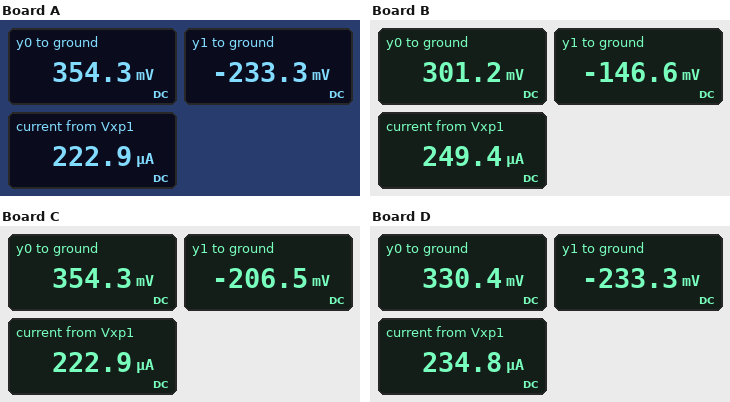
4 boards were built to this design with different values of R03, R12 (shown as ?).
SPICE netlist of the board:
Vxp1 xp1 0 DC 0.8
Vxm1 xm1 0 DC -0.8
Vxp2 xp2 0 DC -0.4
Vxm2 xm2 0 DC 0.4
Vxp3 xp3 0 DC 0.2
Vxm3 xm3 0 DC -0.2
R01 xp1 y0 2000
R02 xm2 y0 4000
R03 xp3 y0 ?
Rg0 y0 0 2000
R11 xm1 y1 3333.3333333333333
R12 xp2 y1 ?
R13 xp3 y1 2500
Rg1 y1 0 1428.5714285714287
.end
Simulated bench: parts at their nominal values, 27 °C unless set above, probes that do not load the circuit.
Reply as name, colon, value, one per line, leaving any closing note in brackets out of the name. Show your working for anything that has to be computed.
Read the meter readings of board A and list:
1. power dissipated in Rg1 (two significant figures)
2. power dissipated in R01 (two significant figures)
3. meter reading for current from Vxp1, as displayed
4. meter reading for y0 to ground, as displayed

power dissipated in Rg1: (0 V - (-233.3 mV))^2 / 1.429 kΩ = 38 µW
power dissipated in R01: (800 mV - 354.3 mV)^2 / 2 kΩ = 99 µW
meter reading for current from Vxp1, as displayed: 222.9 µA
meter reading for y0 to ground, as displayed: 354.3 mV
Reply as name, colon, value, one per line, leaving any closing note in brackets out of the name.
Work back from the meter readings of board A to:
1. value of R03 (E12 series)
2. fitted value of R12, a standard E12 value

value of R03: 2.7 kΩ
fitted value of R12, a standard E12 value: 1 kΩ
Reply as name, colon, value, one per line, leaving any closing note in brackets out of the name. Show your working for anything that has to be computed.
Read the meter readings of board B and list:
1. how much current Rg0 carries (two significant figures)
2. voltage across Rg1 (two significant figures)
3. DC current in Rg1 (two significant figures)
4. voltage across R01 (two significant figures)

how much current Rg0 carries: (301.2 mV) / 2 kΩ = 150 µA
voltage across Rg1: 0 V - (-146.6 mV) = 150 mV
DC current in Rg1: (0 V - (-146.6 mV)) / 1.429 kΩ = 100 µA
voltage across R01: 800 mV - 301.2 mV = 500 mV
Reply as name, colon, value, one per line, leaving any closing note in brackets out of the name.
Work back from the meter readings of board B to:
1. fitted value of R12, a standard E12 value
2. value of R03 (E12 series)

fitted value of R12, a standard E12 value: 5.6 kΩ
value of R03: 820 Ω
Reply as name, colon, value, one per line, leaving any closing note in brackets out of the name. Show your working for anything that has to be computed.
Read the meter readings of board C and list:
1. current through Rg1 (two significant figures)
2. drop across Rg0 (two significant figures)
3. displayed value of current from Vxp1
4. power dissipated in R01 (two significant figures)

current through Rg1: (0 V - (-206.5 mV)) / 1.429 kΩ = 140 µA
drop across Rg0: 354.3 mV = 350 mV
displayed value of current from Vxp1: 222.9 µA
power dissipated in R01: (800 mV - 354.3 mV)^2 / 2 kΩ = 99 µW
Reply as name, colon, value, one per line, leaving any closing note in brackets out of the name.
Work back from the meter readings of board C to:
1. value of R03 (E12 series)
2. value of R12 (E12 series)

value of R03: 2.7 kΩ
value of R12: 1.5 kΩ
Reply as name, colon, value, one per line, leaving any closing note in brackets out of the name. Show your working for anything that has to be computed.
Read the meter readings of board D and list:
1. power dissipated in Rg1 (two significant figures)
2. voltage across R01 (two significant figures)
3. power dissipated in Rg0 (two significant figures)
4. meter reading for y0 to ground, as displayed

power dissipated in Rg1: (0 V - (-233.3 mV))^2 / 1.429 kΩ = 38 µW
voltage across R01: 800 mV - 330.4 mV = 470 mV
power dissipated in Rg0: (330.4 mV)^2 / 2 kΩ = 55 µW
meter reading for y0 to ground, as displayed: 330.4 mV
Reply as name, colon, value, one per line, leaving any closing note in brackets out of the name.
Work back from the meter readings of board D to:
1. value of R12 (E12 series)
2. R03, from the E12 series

value of R12: 1 kΩ
R03, from the E12 series: 1.5 kΩ
